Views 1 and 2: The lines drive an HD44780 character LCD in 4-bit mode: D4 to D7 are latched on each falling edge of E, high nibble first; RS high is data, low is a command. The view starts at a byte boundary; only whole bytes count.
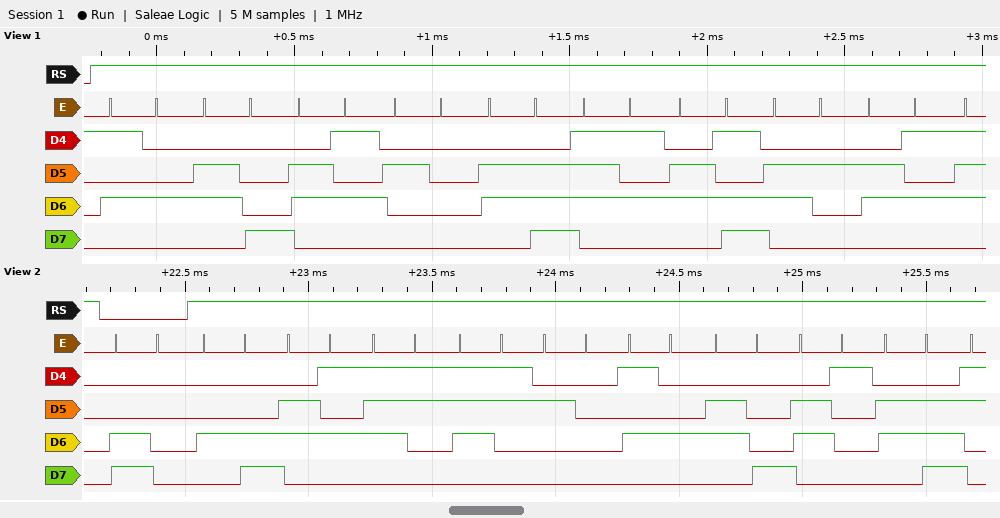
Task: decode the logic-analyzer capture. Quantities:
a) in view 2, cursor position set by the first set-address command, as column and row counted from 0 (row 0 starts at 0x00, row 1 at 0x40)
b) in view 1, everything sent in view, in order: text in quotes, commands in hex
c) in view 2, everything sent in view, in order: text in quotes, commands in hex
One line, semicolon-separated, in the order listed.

column 0, row 1; "The numbe"; 0xC0 "Less Than"
